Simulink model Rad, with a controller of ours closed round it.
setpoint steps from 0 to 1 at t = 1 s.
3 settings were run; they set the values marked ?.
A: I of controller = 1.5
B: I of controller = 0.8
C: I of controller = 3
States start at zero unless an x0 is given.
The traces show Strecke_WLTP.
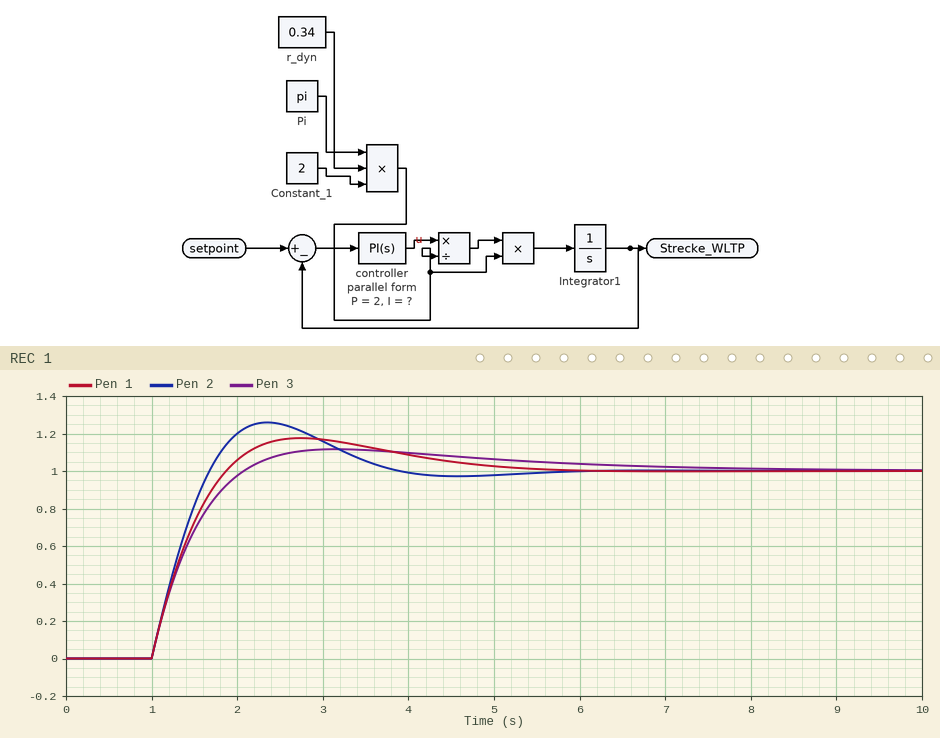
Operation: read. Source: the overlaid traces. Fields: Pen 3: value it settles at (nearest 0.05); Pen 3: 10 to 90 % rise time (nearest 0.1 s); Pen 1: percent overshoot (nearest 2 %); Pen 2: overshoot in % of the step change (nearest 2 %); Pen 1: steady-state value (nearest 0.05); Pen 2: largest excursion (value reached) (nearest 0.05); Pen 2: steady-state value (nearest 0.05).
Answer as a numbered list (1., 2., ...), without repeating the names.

1. 1.00
2. 0.8 s
3. 18 %
4. 26 %
5. 1.00
6. 1.25
7. 1.00
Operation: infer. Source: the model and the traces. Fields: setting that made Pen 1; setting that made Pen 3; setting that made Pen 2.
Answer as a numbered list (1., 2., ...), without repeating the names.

1. A
2. B
3. C
